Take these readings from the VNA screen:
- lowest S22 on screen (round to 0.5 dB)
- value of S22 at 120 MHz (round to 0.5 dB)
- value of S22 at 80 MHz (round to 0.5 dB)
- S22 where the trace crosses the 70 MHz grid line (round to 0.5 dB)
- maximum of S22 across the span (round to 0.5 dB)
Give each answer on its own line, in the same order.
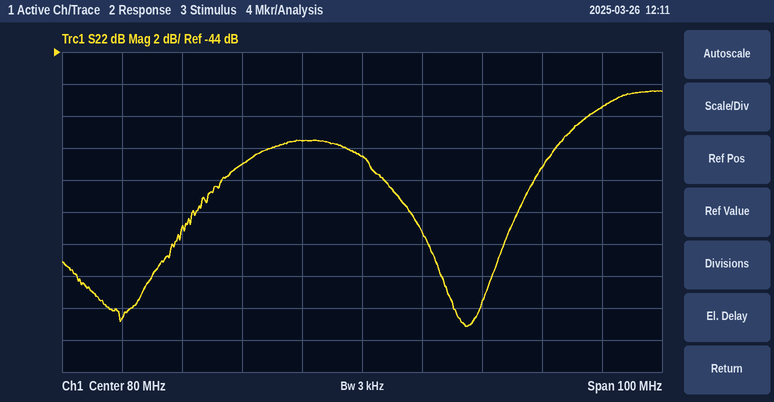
-61.0 dB
-47.5 dB
-50.5 dB
-49.5 dB
-46.5 dB
